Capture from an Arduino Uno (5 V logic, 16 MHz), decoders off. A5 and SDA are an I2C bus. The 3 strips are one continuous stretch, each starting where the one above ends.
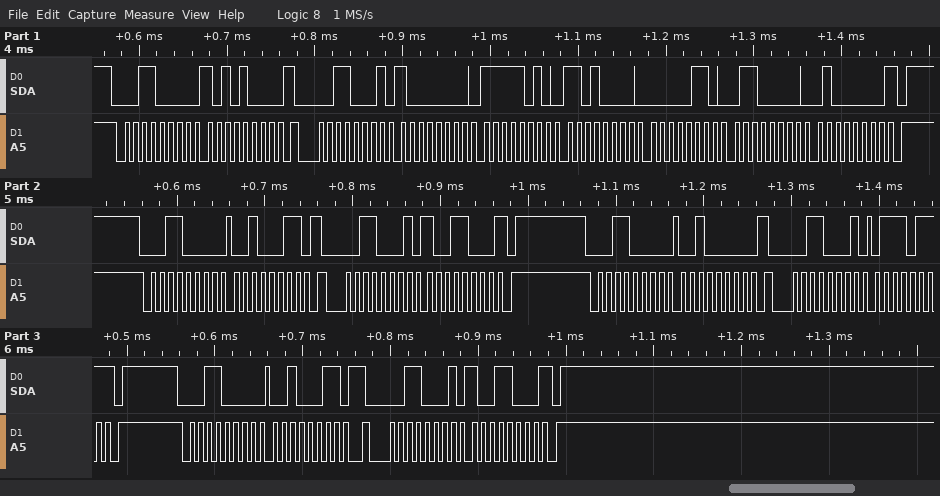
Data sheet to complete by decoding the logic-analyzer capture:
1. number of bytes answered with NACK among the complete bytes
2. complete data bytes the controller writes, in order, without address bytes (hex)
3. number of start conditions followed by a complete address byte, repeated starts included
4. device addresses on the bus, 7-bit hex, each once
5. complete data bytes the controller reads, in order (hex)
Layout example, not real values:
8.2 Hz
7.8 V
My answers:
4
A8 23 20 23
8
0x18
80 FA D0 06 60 40 98 77 98
